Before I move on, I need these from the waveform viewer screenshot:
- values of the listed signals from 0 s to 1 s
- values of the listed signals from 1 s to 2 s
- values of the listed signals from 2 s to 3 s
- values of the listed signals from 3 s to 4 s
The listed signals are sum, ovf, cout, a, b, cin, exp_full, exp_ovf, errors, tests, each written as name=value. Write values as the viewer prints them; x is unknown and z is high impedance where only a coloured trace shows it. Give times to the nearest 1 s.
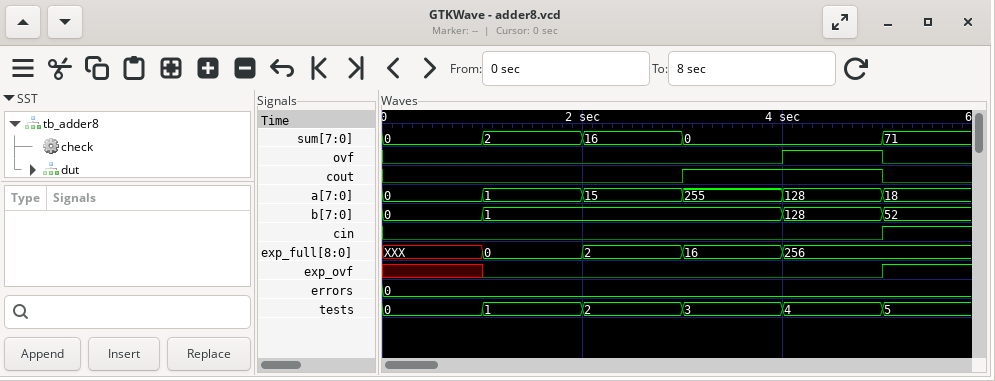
sum=0, ovf=0, cout=0, a=0, b=0, cin=0, exp_full=XXX, exp_ovf=x, errors=0, tests=0
sum=2, ovf=0, cout=0, a=1, b=1, cin=0, exp_full=0, exp_ovf=0, errors=0, tests=1
sum=16, ovf=0, cout=0, a=15, b=1, cin=0, exp_full=2, exp_ovf=0, errors=0, tests=2
sum=0, ovf=0, cout=1, a=255, b=1, cin=0, exp_full=16, exp_ovf=0, errors=0, tests=3
